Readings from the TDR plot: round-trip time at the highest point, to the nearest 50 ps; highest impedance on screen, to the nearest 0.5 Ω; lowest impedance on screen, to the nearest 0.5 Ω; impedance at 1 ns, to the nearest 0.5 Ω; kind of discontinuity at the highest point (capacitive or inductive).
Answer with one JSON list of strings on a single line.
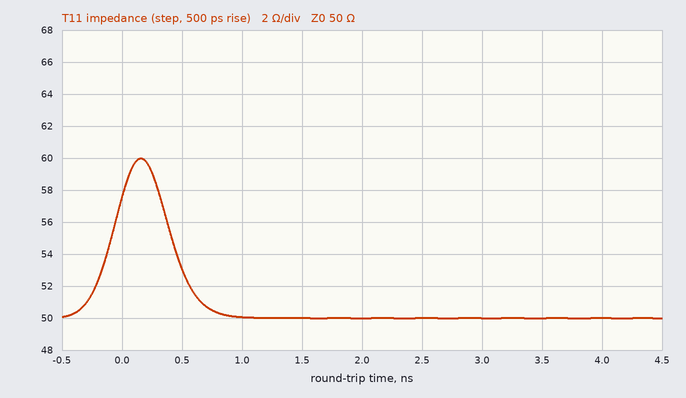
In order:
["150 ps", "60.0 Ω", "50.0 Ω", "50.0 Ω", "inductive"]
